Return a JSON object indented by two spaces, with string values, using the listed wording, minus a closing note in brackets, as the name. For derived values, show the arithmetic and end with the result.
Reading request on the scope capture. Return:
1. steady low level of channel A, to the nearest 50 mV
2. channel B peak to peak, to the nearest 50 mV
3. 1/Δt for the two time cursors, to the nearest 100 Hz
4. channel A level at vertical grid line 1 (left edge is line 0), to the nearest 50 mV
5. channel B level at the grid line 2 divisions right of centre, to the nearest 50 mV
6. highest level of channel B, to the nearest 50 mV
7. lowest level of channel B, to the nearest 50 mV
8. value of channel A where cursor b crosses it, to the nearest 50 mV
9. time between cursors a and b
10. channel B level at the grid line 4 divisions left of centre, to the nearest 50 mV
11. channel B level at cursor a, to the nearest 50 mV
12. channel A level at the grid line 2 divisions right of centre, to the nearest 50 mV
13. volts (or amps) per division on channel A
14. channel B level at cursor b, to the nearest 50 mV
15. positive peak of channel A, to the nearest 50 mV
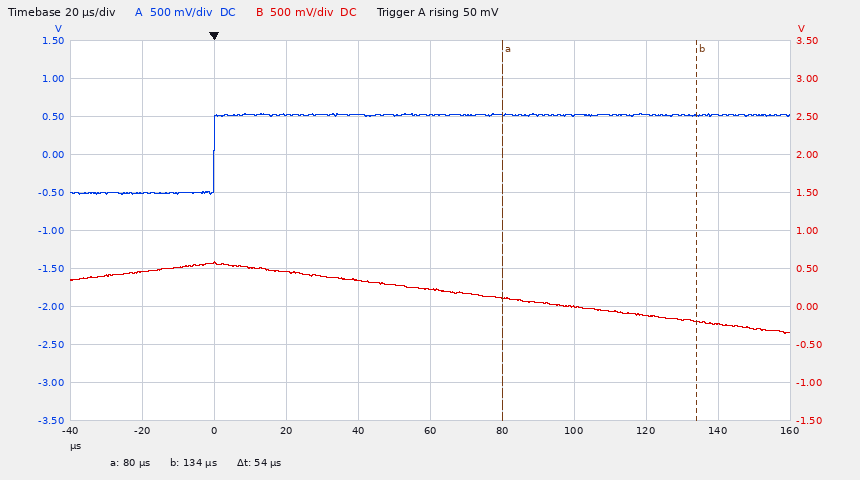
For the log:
{
  "steady low level of channel A, to the nearest 50 mV": "-500 mV",
  "channel B peak to peak, to the nearest 50 mV": "600 mV − (-350 mV) = 950 mV",
  "1/Δt for the two time cursors, to the nearest 100 Hz": "1 / 54 µs ≈ 18.5 kHz",
  "channel A level at vertical grid line 1 (left edge is line 0), to the nearest 50 mV": "-500 mV",
  "channel B level at the grid line 2 divisions right of centre, to the nearest 50 mV": "0 mV",
  "highest level of channel B, to the nearest 50 mV": "600 mV",
  "lowest level of channel B, to the nearest 50 mV": "-350 mV",
  "value of channel A where cursor b crosses it, to the nearest 50 mV": "500 mV",
  "time between cursors a and b": "54 µs",
  "channel B level at the grid line 4 divisions left of centre, to the nearest 50 mV": "450 mV",
  "channel B level at cursor a, to the nearest 50 mV": "100 mV",
  "channel A level at the grid line 2 divisions right of centre, to the nearest 50 mV": "500 mV",
  "volts (or amps) per division on channel A": "500 mV",
  "channel B level at cursor b, to the nearest 50 mV": "-200 mV",
  "positive peak of channel A, to the nearest 50 mV": "550 mV"
}
